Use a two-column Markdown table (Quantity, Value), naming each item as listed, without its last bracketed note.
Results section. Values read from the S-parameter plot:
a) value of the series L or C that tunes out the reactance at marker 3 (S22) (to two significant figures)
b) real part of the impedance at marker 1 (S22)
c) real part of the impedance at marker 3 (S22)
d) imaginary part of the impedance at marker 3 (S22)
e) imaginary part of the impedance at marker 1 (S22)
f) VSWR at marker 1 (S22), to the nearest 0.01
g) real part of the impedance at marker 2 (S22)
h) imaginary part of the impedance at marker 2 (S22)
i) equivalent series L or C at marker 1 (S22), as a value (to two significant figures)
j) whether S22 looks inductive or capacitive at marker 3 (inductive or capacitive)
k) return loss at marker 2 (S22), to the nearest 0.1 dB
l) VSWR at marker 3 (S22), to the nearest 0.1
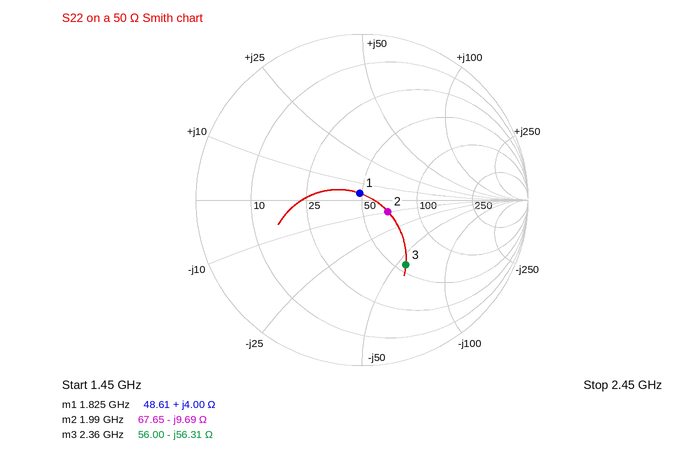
| Quantity | Value |
|---|---|
| value of the series L or C that tunes out the reactance at marker 3 (S22) | 3.8 nH |
| real part of the impedance at marker 1 | 48.61 Ω |
| real part of the impedance at marker 3 | 56.00 Ω |
| imaginary part of the impedance at marker 3 | -56.31 Ω |
| imaginary part of the impedance at marker 1 | +4.00 Ω |
| VSWR at marker 1 (S22), to the nearest 0.01 | 1.09 |
| real part of the impedance at marker 2 | 67.65 Ω |
| imaginary part of the impedance at marker 2 | -9.69 Ω |
| equivalent series L or C at marker 1 (S22), as a value | 350 pH |
| whether S22 looks inductive or capacitive at marker 3 | capacitive |
| return loss at marker 2 (S22), to the nearest 0.1 dB | 15.4 dB |
| VSWR at marker 3 (S22), to the nearest 0.1 | 2.8 |
